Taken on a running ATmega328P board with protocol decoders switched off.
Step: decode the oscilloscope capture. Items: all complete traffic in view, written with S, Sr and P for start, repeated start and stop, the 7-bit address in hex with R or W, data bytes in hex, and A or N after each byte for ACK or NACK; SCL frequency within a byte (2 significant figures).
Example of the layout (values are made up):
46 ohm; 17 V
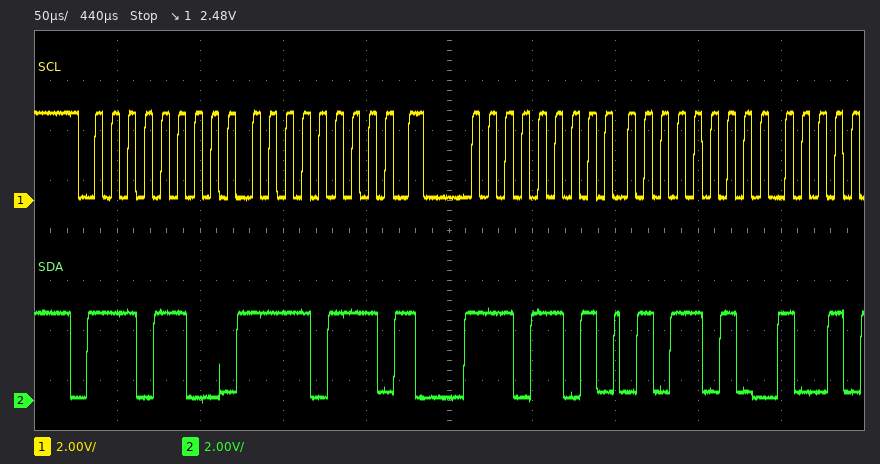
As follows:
S 76W A F7 A Sr 76R A 5A A; 100 kHz
